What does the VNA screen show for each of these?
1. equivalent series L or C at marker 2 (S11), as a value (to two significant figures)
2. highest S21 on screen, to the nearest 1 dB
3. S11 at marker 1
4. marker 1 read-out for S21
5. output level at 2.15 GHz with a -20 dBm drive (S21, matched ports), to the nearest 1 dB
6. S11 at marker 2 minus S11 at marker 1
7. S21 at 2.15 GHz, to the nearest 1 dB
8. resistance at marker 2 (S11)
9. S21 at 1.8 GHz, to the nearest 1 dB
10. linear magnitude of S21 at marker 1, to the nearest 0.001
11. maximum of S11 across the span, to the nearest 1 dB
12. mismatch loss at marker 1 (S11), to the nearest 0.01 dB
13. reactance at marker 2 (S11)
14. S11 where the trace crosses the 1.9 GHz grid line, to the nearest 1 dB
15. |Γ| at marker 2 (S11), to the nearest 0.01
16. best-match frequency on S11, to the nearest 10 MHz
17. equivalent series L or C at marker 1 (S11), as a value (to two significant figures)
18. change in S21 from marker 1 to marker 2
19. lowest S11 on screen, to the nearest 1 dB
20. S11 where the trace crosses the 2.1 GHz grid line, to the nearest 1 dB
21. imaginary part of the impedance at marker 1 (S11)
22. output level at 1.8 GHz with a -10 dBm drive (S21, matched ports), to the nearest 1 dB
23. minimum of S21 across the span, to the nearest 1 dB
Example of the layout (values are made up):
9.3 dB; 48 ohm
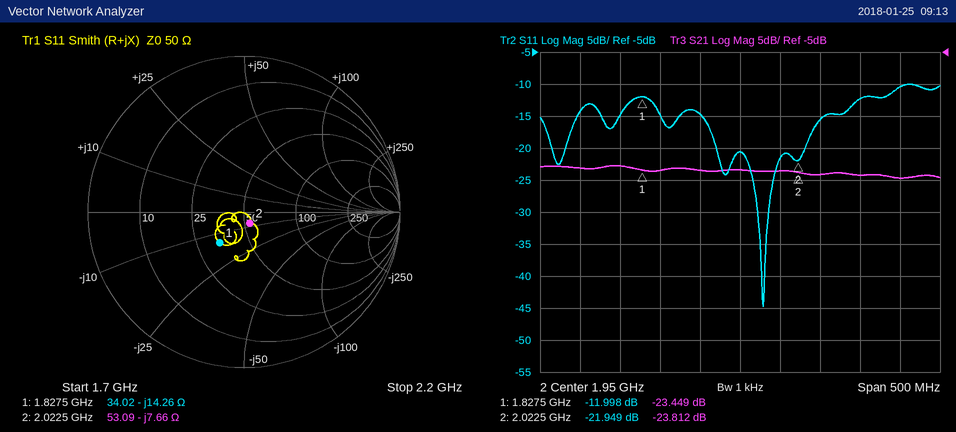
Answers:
10 pF; -23 dB; -11.998 dB; -23.449 dB; -45 dBm; -9.951 dB; -25 dB; 53.09 Ω; -23 dB; 0.067; -10 dB; 0.28 dB; -7.66 Ω; -15 dB; 0.08; 1.98 GHz; 6.1 pF; -0.363 dB; -45 dB; -12 dB; -14.26 Ω; -33 dBm; -25 dB
